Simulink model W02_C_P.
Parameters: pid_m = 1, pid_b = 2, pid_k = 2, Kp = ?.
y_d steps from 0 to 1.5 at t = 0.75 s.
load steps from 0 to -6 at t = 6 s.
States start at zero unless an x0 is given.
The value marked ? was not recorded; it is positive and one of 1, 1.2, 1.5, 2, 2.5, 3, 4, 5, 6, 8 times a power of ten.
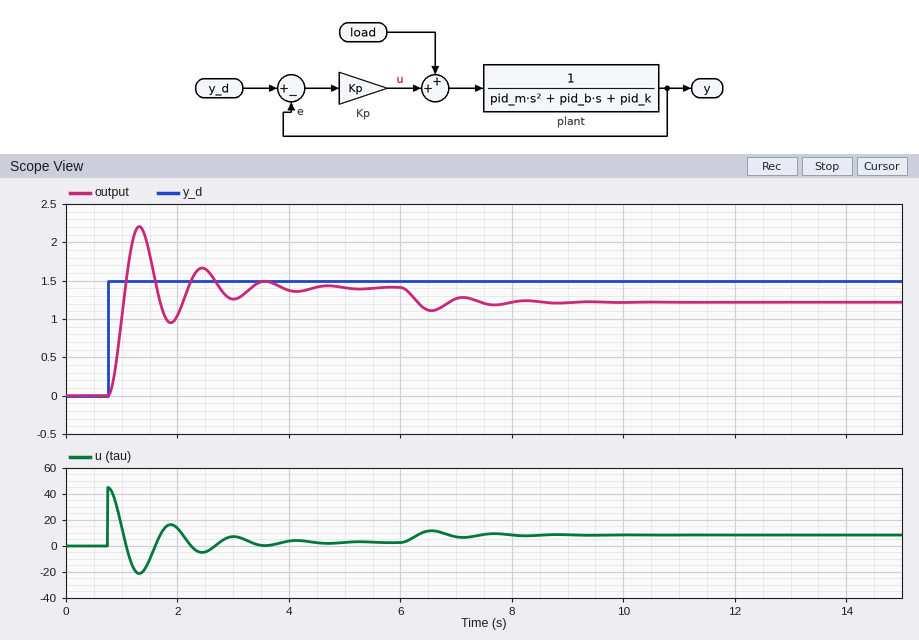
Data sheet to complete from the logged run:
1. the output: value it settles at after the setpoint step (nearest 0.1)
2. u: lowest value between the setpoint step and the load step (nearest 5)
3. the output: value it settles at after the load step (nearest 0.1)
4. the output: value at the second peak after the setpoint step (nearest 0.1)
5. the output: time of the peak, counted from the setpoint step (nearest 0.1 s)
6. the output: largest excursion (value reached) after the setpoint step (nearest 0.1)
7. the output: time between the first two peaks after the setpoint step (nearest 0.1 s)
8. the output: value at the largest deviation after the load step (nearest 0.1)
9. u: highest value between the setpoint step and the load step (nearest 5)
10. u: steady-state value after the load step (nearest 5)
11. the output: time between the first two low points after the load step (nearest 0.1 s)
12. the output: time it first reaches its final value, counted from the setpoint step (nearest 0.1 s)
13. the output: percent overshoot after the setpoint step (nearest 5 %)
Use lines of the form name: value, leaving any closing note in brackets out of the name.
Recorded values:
the output: value it settles at after the setpoint step: 1.4
u: lowest value between the setpoint step and the load step: -20
the output: value it settles at after the load step: 1.2
the output: value at the second peak after the setpoint step: 1.7
the output: time of the peak, counted from the setpoint step: 0.6 s
the output: largest excursion (value reached) after the setpoint step: 2.2
the output: time between the first two peaks after the setpoint step: 1.1 s
the output: value at the largest deviation after the load step: 1.1
u: highest value between the setpoint step and the load step: 45
u: steady-state value after the load step: 10
the output: time between the first two low points after the load step: 1.1 s
the output: time it first reaches its final value, counted from the setpoint step: 0.3 s
the output: percent overshoot after the setpoint step: 55 %
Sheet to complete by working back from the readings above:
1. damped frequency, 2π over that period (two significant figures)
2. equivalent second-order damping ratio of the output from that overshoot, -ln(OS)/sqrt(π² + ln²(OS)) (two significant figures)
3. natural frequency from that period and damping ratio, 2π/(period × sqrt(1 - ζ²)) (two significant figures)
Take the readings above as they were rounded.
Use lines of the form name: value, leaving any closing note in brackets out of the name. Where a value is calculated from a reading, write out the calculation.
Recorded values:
damped frequency, 2π over that period: 2π / 1.1 = 5.7 rad/s
equivalent second-order damping ratio of the output from that overshoot, -ln(OS)/sqrt(π² + ln²(OS)): ln(0.55) = -0.598; 0.598 / sqrt(9.870 + 0.357) = 0.19
natural frequency from that period and damping ratio, 2π/(period × sqrt(1 - ζ²)): 2π / (1.1 × sqrt(1 - 0.19²)) = 5.8 rad/s
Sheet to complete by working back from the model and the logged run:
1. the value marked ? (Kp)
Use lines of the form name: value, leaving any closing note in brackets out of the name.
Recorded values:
the value marked ?: 30
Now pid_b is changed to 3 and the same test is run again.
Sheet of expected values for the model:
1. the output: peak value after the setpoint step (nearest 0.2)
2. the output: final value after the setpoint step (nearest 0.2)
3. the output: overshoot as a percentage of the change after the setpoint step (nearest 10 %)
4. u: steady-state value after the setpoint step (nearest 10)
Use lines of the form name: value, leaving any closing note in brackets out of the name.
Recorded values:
the output: peak value after the setpoint step: 2.0
the output: final value after the setpoint step: 1.4
the output: overshoot as a percentage of the change after the setpoint step: 40 %
u: steady-state value after the setpoint step: 0
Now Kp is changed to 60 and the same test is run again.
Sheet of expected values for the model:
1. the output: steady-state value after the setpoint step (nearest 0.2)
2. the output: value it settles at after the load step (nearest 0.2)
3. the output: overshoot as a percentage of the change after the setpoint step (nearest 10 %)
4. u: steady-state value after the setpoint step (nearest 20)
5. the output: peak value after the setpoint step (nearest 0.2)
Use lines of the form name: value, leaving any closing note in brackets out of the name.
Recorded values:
the output: steady-state value after the setpoint step: 1.4
the output: value it settles at after the load step: 1.4
the output: overshoot as a percentage of the change after the setpoint step: 70 %
u: steady-state value after the setpoint step: 0
the output: peak value after the setpoint step: 2.4
